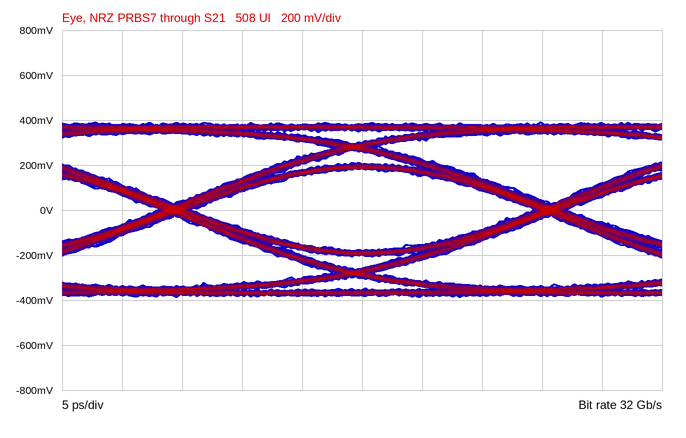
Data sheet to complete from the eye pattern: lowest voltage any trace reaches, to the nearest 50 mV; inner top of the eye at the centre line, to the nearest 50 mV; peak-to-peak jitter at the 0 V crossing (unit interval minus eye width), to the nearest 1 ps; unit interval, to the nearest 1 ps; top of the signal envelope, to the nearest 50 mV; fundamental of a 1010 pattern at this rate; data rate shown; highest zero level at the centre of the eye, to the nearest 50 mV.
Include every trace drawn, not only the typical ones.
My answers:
-400 mV
200 mV
3 ps
31 ps
400 mV
16 GHz
32 Gb/s
-200 mV
